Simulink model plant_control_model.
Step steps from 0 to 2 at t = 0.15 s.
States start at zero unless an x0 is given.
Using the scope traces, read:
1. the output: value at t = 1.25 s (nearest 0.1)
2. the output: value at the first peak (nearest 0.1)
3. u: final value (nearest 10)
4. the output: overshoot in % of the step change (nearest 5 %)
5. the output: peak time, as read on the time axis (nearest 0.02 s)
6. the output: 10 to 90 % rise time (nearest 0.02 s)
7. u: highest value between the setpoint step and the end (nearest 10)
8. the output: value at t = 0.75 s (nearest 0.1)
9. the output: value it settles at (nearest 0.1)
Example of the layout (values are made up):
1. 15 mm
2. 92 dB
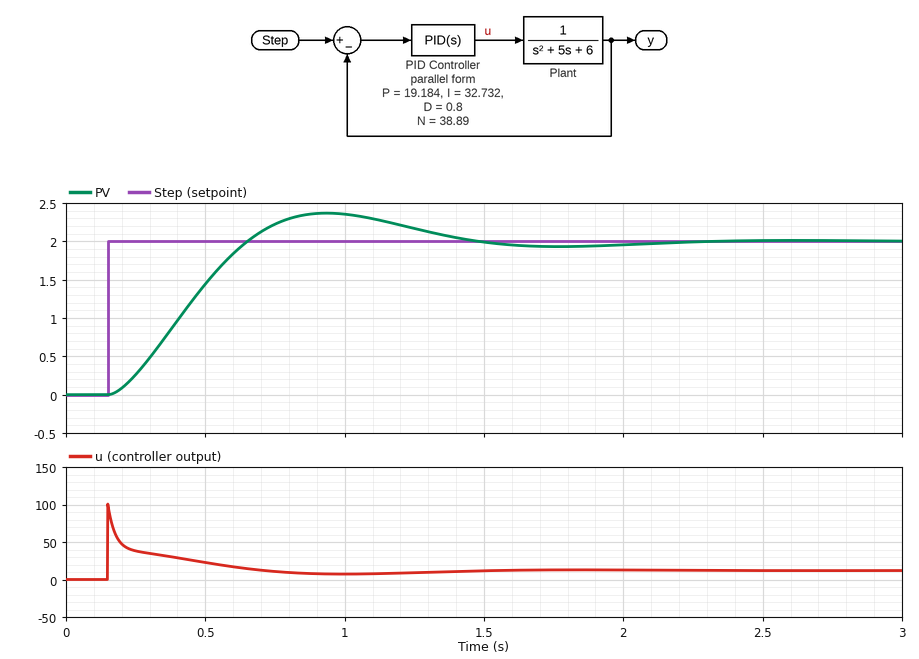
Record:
1. 2.2
2. 2.4
3. 10
4. 20 %
5. 0.94 s
6. 0.36 s
7. 100
8. 2.2
9. 2.0
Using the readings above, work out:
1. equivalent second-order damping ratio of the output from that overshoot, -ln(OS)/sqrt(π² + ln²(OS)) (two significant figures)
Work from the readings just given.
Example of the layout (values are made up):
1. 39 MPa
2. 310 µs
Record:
1. 0.46
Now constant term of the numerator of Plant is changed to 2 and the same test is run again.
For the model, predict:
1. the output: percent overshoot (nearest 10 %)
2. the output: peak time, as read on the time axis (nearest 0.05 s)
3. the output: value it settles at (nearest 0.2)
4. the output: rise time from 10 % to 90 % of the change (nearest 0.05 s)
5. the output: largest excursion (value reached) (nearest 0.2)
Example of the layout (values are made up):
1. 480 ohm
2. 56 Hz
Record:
1. 30 %
2. 0.65 s
3. 2.0
4. 0.20 s
5. 2.6
